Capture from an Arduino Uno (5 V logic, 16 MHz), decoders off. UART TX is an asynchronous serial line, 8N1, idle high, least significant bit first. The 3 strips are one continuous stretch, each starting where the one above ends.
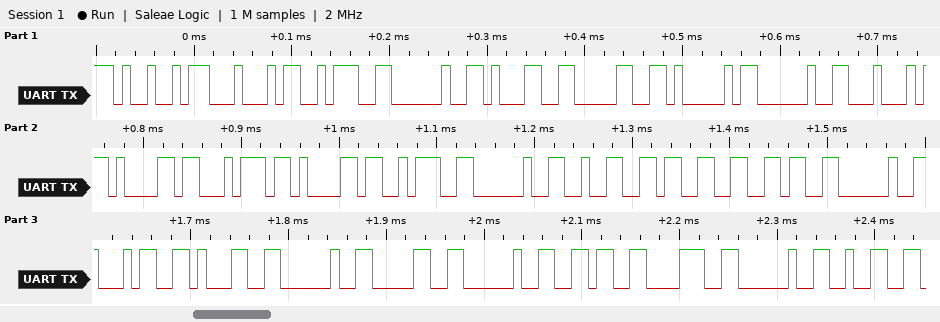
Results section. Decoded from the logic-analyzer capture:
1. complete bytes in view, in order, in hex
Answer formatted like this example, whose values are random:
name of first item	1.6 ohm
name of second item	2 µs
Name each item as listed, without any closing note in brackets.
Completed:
complete bytes in view, in order, in hex	49 44 3A 20 31 30 41 20 44 61 74 61 3A 20 32 33 36 20 34 31 20 30 20 36 38 20 32
